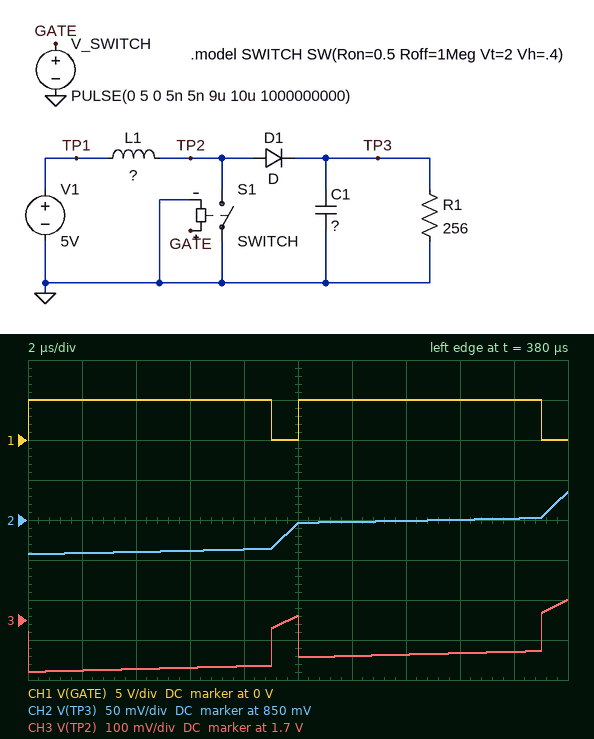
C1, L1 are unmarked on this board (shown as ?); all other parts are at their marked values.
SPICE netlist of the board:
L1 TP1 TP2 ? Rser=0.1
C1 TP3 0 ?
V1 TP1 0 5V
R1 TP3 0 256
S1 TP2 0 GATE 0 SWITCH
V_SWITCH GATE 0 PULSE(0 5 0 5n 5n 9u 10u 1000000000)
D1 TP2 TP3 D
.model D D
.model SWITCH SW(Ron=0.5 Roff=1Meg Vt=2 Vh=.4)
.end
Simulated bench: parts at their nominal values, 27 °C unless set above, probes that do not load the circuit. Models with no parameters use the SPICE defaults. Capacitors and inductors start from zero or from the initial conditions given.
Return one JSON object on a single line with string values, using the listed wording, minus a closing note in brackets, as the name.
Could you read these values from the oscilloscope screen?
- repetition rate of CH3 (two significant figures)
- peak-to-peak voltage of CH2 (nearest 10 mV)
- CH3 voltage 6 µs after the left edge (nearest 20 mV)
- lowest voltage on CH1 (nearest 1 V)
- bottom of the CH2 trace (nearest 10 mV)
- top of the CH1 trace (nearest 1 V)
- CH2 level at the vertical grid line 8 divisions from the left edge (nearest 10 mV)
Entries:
{"repetition rate of CH3": "100 kHz", "peak-to-peak voltage of CH2": "80 mV", "CH3 voltage 6 µs after the left edge": "1.58 V", "lowest voltage on CH1": "0 V", "bottom of the CH2 trace": "810 mV", "top of the CH1 trace": "5 V", "CH2 level at the vertical grid line 8 divisions from the left edge": "850 mV"}
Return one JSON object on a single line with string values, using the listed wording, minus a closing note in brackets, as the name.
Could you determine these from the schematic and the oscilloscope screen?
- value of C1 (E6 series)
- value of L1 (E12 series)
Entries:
{"value of C1": "100 µF", "value of L1": "470 µH"}
